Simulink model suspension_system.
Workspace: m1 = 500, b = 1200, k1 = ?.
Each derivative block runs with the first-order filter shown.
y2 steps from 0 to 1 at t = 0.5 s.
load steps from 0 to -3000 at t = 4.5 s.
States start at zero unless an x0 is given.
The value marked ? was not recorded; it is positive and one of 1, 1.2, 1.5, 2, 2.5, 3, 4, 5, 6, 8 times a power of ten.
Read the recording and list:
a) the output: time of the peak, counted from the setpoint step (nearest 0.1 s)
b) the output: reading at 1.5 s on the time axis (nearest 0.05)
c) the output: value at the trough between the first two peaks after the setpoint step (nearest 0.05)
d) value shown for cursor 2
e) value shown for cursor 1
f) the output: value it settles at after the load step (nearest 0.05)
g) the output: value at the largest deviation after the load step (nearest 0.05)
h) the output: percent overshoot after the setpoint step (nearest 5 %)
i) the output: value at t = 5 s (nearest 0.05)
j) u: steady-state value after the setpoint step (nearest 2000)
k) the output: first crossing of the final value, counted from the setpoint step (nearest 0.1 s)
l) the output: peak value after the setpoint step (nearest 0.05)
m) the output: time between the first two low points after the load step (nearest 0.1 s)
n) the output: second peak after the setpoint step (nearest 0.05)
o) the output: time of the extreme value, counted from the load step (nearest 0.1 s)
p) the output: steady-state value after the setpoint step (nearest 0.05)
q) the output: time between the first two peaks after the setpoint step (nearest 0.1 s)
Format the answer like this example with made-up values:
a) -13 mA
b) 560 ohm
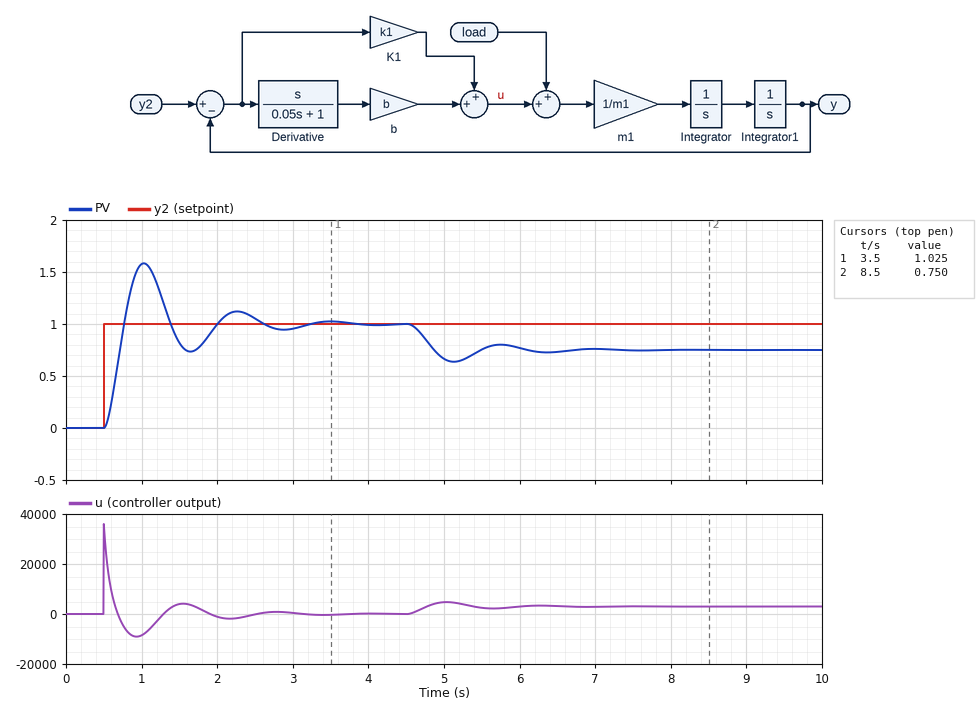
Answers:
a) 0.5 s
b) 0.80
c) 0.75
d) 0.750
e) 1.025
f) 0.75
g) 0.65
h) 60 %
i) 0.65
j) 0
k) 0.3 s
l) 1.60
m) 1.2 s
n) 1.10
o) 0.6 s
p) 1.00
q) 1.2 s
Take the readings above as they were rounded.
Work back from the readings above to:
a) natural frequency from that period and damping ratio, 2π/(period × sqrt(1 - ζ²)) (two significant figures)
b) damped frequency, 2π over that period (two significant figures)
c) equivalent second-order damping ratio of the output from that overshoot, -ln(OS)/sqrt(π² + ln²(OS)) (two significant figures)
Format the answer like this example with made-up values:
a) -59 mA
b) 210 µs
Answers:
a) 5.3 rad/s
b) 5.2 rad/s
c) 0.16
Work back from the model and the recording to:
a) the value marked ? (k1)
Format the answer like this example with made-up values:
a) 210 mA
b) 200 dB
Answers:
a) 12000
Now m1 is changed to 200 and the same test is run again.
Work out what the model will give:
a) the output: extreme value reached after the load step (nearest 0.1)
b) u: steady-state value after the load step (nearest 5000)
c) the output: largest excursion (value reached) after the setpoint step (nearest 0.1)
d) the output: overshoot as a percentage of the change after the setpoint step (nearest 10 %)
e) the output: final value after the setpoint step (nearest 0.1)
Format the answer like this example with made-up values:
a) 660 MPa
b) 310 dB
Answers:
a) 0.7
b) 5000
c) 1.5
d) 50 %
e) 1.0
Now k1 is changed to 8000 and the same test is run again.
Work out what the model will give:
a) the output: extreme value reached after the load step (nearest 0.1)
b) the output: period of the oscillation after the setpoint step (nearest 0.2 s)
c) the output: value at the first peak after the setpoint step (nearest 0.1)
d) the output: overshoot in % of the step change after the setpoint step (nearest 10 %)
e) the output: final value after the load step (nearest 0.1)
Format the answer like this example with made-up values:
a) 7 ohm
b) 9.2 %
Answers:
a) 0.5
b) 1.6 s
c) 1.5
d) 50 %
e) 0.6
